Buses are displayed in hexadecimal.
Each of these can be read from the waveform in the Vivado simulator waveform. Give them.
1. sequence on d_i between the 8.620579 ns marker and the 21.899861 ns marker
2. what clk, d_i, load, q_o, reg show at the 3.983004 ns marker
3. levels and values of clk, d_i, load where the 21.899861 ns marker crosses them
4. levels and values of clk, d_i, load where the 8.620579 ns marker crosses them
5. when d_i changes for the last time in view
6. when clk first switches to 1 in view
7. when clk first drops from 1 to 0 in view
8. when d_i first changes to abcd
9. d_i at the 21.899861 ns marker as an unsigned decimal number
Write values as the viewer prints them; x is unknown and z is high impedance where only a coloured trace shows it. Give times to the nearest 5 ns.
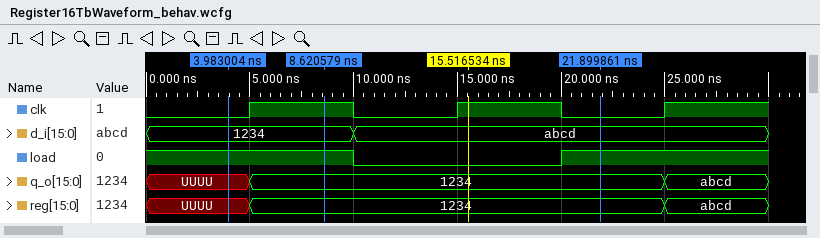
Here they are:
1234, abcd
clk=0, d_i=1234, load=1, q_o=UUUU, reg=UUUU
clk=0, d_i=abcd, load=1
clk=1, d_i=1234, load=1
10 ns
5 ns
10 ns
10 ns
43981
